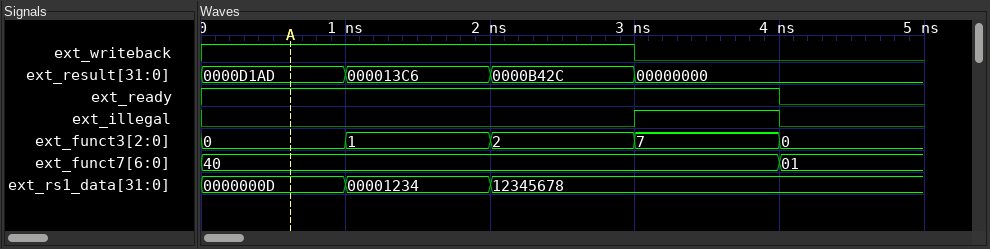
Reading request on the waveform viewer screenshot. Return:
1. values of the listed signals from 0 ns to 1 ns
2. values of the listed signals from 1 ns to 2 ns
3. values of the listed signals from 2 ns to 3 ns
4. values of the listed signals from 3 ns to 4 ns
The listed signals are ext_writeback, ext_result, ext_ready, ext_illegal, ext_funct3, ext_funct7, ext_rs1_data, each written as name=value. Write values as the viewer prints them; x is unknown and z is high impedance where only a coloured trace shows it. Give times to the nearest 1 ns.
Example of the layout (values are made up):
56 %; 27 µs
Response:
ext_writeback=1, ext_result=0000D1AD, ext_ready=1, ext_illegal=0, ext_funct3=0, ext_funct7=40, ext_rs1_data=0000000D; ext_writeback=1, ext_result=000013C6, ext_ready=1, ext_illegal=0, ext_funct3=1, ext_funct7=40, ext_rs1_data=00001234; ext_writeback=1, ext_result=0000B42C, ext_ready=1, ext_illegal=0, ext_funct3=2, ext_funct7=40, ext_rs1_data=12345678; ext_writeback=0, ext_result=00000000, ext_ready=1, ext_illegal=1, ext_funct3=7, ext_funct7=40, ext_rs1_data=12345678
